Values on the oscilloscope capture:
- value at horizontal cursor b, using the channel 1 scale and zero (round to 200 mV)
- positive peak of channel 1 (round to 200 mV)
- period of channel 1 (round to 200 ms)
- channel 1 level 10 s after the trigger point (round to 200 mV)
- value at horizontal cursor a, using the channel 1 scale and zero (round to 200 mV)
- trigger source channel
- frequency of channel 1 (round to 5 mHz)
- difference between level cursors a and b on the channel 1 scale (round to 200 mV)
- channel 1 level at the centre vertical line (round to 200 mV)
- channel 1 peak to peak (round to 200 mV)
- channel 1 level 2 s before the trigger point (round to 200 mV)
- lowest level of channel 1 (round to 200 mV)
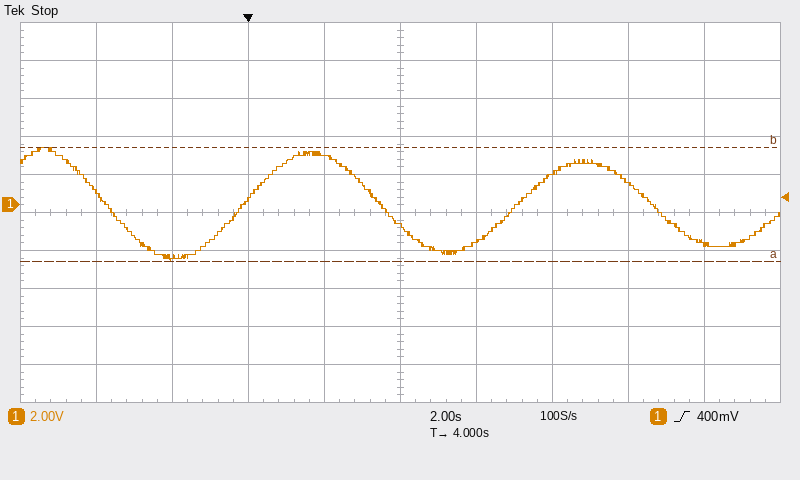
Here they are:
3.0 V
3.0 V
7.2 s
1.2 V
-3.0 V
channel 1
140 mHz
6.0 V
-1.2 V
6.0 V
-2.8 V
-3.0 V
